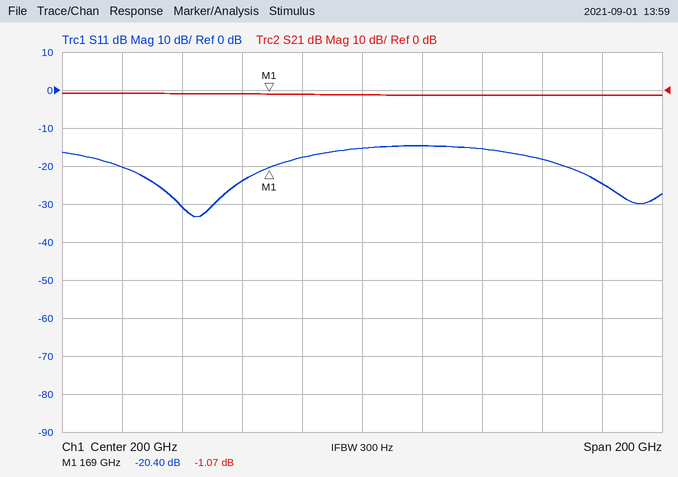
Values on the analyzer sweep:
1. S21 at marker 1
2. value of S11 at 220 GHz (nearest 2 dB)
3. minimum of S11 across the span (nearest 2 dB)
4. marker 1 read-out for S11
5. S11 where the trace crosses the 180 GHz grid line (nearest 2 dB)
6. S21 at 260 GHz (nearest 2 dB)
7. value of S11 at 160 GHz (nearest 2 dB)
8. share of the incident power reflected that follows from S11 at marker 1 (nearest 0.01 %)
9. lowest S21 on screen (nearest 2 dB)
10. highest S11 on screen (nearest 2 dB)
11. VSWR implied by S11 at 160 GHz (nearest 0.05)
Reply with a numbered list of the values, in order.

1. -1.07 dB
2. -14 dB
3. -34 dB
4. -20.40 dB
5. -18 dB
6. -2 dB
7. -24 dB
8. 0.91 %
9. -2 dB
10. -14 dB
11. 1.15
